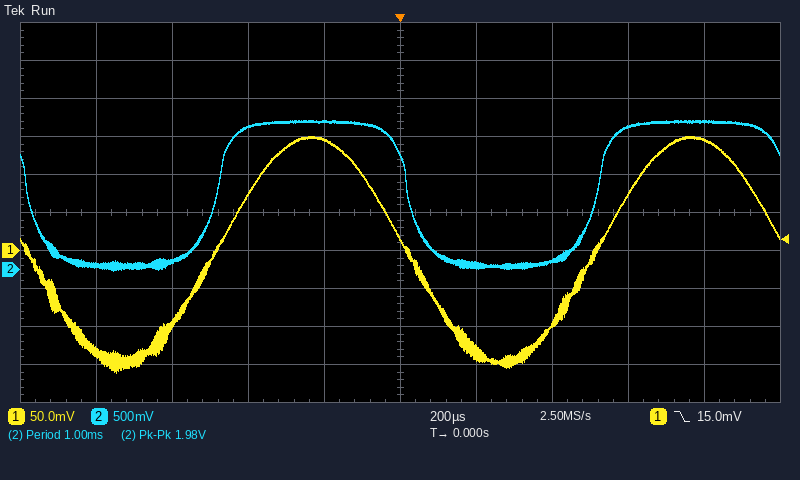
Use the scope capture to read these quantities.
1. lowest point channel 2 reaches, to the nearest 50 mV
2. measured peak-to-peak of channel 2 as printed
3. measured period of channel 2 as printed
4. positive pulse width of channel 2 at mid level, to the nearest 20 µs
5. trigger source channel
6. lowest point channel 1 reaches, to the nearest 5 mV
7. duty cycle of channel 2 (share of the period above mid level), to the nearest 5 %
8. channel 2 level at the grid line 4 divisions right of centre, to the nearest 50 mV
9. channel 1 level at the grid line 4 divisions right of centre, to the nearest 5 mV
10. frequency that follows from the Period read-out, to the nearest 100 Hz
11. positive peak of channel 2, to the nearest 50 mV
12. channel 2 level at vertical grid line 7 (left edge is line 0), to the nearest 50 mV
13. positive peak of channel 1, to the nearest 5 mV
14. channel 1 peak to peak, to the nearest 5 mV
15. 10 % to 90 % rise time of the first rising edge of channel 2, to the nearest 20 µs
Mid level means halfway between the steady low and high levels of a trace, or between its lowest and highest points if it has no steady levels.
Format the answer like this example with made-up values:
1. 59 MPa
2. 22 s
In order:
1. 0 mV
2. 1.98 V
3. 1.00 ms
4. 500 µs
5. channel 1
6. -160 mV
7. 50 %
8. 1.95 V
9. 145 mV
10. 1.0 kHz
11. 1.95 V
12. 100 mV
13. 150 mV
14. 310 mV
15. 120 µs
